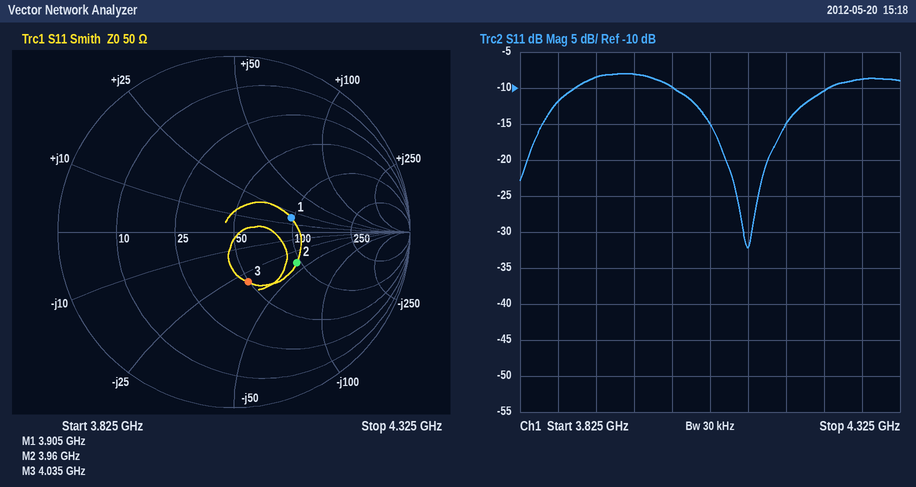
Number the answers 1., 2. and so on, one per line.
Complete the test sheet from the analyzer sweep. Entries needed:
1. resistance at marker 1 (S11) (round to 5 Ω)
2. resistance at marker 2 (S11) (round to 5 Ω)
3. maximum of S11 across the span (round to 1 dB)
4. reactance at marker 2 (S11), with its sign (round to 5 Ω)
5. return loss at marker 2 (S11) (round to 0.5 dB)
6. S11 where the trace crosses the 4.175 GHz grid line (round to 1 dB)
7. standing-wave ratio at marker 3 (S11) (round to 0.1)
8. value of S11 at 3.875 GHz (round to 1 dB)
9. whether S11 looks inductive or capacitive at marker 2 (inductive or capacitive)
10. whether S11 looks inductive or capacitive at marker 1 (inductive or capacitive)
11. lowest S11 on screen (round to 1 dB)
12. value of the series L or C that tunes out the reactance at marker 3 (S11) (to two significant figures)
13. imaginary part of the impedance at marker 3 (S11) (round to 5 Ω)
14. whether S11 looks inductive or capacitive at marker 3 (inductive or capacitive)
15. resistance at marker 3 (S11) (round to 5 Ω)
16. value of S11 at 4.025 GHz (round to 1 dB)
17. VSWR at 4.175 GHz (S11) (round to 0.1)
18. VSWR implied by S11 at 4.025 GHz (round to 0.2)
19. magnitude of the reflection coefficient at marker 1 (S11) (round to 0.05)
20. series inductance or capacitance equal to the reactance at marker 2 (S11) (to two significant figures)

1. 95 Ω
2. 95 Ω
3. -8 dB
4. -40 Ω
5. 8.0 dB
6. -15 dB
7. 1.8
8. -12 dB
9. capacitive
10. inductive
11. -32 dB
12. 1.2 nH
13. -30 Ω
14. capacitive
15. 50 Ω
16. -10 dB
17. 1.4
18. 2.0
19. 0.35
20. 1.0 pF
